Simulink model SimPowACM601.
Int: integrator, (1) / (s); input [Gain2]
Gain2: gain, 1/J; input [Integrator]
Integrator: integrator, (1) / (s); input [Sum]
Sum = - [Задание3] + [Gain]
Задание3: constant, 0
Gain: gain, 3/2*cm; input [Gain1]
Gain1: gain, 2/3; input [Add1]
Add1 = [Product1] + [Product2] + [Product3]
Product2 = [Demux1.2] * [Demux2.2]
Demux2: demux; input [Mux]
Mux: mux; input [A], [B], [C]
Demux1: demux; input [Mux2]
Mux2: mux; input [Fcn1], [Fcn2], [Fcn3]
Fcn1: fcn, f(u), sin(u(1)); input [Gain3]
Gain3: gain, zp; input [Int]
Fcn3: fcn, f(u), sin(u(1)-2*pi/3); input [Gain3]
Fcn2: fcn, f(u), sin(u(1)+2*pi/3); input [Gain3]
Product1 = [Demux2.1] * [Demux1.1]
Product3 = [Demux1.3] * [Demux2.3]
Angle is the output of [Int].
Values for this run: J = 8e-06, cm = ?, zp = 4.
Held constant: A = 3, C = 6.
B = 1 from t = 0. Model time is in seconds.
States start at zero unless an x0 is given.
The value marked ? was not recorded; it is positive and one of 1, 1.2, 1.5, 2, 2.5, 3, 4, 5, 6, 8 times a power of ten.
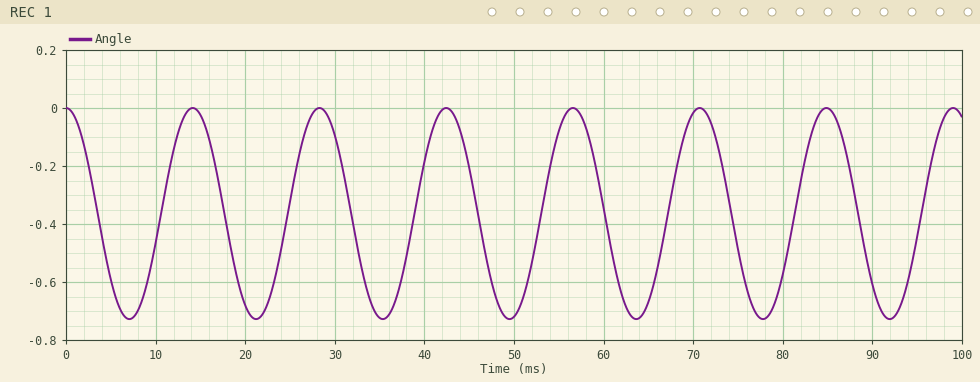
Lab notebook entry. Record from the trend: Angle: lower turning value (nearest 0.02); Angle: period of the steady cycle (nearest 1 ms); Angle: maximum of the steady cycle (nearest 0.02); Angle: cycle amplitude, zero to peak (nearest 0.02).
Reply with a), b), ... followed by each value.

a) -0.72
b) 14 ms
c) 0.00
d) 0.36
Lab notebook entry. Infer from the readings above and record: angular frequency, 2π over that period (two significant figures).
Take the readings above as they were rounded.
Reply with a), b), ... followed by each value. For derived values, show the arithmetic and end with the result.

a) 2π / 14 = 0.45 rad/ms
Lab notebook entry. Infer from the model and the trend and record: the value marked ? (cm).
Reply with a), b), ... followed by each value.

a) 0.12
